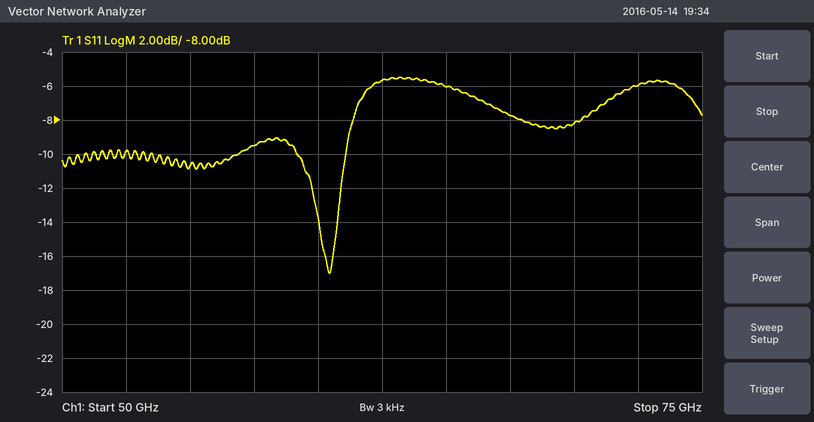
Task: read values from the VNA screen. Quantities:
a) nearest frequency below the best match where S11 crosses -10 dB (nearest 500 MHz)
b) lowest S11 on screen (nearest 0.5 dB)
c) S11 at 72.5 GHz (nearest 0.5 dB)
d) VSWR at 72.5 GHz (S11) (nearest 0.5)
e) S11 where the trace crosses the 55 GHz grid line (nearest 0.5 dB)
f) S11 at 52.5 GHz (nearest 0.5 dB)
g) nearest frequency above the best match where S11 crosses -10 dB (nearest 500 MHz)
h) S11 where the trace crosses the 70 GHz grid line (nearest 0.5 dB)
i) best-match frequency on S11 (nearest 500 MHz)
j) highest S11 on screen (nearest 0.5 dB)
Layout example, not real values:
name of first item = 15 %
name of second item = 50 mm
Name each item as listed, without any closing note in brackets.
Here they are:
nearest frequency below the best match where S11 crosses -10 dB = 59.0 GHz
lowest S11 on screen = -17.0 dB
S11 at 72.5 GHz = -6.0 dB
VSWR at 72.5 GHz (S11) = 3.0
S11 where the trace crosses the 55 GHz grid line = -10.5 dB
S11 at 52.5 GHz = -10.0 dB
nearest frequency above the best match where S11 crosses -10 dB = 61.0 GHz
S11 where the trace crosses the 70 GHz grid line = -8.0 dB
best-match frequency on S11 = 60.5 GHz
highest S11 on screen = -5.5 dB
